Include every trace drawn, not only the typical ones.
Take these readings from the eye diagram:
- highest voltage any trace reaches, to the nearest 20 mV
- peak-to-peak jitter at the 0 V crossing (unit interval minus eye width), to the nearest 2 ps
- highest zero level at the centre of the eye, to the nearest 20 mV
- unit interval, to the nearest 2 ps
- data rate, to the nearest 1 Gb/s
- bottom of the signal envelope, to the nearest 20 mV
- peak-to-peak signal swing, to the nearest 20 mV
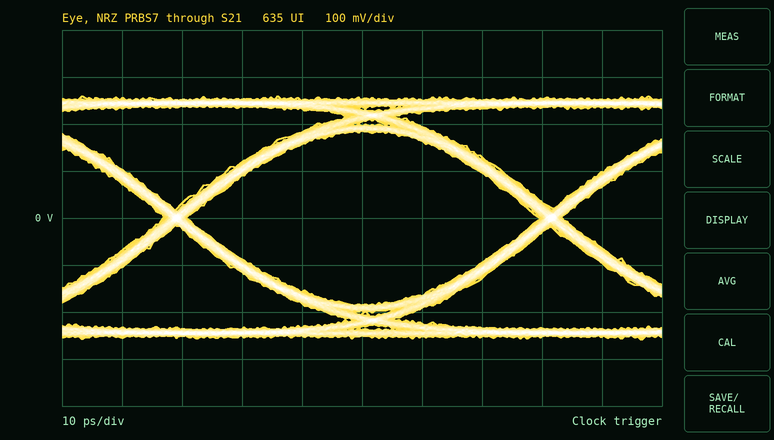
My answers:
260 mV
4 ps
-180 mV
62 ps
16 Gb/s
-260 mV
520 mV
